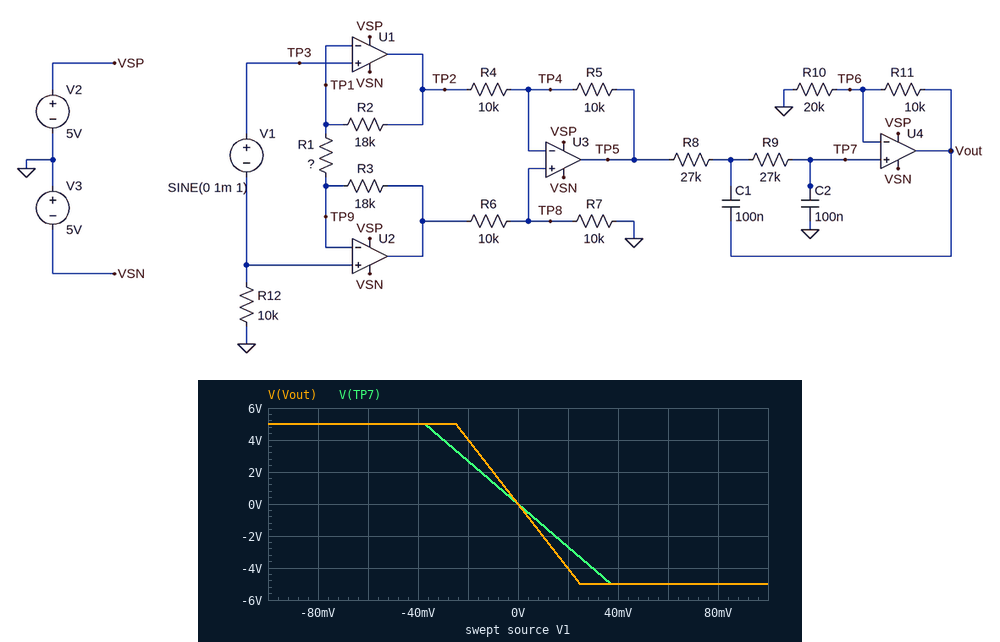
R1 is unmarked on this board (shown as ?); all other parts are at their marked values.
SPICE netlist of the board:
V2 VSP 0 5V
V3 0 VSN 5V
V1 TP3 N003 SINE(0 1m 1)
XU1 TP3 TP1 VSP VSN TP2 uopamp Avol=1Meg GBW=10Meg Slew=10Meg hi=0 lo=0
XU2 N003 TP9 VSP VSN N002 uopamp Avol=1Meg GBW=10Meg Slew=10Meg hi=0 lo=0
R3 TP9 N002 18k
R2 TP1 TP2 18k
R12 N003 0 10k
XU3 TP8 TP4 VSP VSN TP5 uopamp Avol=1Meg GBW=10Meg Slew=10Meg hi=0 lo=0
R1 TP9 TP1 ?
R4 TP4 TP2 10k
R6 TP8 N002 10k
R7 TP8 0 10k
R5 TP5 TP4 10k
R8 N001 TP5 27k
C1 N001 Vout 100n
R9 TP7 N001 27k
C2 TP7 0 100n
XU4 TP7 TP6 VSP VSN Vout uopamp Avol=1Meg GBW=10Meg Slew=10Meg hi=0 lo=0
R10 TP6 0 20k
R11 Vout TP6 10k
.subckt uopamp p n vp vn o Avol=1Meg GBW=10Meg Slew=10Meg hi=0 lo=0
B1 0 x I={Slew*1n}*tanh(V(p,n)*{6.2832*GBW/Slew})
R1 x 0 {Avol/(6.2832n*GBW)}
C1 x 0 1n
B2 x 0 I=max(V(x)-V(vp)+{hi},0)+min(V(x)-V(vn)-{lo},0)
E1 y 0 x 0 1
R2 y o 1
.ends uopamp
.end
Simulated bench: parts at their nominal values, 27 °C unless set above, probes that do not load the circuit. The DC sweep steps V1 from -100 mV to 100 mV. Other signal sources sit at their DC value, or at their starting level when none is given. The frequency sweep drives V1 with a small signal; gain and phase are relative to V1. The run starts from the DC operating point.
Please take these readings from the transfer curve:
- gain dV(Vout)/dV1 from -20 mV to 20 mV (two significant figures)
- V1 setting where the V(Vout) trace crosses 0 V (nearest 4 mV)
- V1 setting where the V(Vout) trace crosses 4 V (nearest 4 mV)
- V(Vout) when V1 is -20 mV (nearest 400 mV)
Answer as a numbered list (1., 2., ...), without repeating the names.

1. -200 V/V
2. 0 V
3. -20 mV
4. 4.0 V
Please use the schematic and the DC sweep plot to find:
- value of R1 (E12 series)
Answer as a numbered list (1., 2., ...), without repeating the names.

1. 270 Ω
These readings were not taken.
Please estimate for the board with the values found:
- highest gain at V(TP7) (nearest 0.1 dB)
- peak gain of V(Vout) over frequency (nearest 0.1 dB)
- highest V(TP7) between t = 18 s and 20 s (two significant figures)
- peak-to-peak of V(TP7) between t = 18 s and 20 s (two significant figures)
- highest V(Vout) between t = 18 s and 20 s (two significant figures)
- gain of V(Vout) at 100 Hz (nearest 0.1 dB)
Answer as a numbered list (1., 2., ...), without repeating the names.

1. 42.6 dB
2. 46.1 dB
3. 130 mV
4. 270 mV
5. 200 mV
6. 36.1 dB
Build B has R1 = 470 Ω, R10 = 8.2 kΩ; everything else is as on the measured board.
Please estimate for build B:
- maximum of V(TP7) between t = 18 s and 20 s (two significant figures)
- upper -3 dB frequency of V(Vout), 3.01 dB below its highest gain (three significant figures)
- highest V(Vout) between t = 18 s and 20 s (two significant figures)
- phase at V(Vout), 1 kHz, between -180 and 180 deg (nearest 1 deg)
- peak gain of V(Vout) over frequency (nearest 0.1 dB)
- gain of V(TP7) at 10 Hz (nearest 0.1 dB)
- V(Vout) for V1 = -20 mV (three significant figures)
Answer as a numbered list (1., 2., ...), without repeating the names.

1. 78 mV
2. 70.1 Hz
3. 170 mV
4. 2 deg
5. 47.6 dB
6. 38.0 dB
7. 3.44 V
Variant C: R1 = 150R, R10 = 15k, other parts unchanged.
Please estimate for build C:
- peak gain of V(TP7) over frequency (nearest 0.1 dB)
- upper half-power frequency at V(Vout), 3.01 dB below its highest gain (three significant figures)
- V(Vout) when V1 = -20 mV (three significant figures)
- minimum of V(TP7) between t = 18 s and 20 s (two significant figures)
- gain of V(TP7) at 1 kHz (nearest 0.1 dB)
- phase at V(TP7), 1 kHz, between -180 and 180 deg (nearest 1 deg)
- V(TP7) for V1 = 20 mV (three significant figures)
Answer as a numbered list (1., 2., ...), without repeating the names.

1. 47.7 dB
2. 62.0 Hz
3. 5.01 V
4. -240 mV
5. -1.5 dB
6. 3 deg
7. -4.82 V
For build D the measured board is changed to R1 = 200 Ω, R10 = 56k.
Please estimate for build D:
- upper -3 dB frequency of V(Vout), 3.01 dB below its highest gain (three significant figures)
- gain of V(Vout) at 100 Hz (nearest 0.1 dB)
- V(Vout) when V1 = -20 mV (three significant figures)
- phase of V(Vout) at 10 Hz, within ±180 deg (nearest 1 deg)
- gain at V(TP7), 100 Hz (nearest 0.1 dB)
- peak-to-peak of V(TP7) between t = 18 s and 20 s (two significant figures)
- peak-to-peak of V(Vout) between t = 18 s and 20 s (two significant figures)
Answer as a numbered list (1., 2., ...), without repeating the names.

1. 43.3 Hz
2. 35.4 dB
3. 4.27 V
4. 162 deg
5. 34.0 dB
6. 360 mV
7. 430 mV
